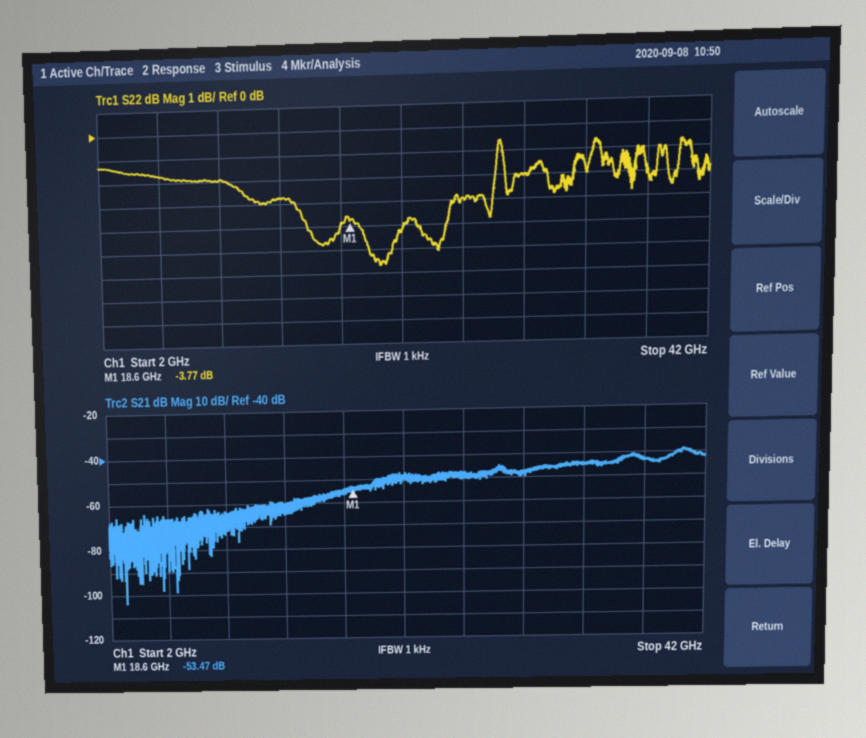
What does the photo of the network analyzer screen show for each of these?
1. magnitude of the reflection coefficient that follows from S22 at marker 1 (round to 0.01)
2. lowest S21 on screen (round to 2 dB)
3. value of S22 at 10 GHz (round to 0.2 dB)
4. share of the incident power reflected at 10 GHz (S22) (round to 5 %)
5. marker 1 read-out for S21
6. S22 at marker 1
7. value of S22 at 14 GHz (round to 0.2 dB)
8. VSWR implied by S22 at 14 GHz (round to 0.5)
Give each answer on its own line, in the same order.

0.65
-104 dB
-2.0 dB
65 %
-53.47 dB
-3.77 dB
-2.8 dB
6.5
